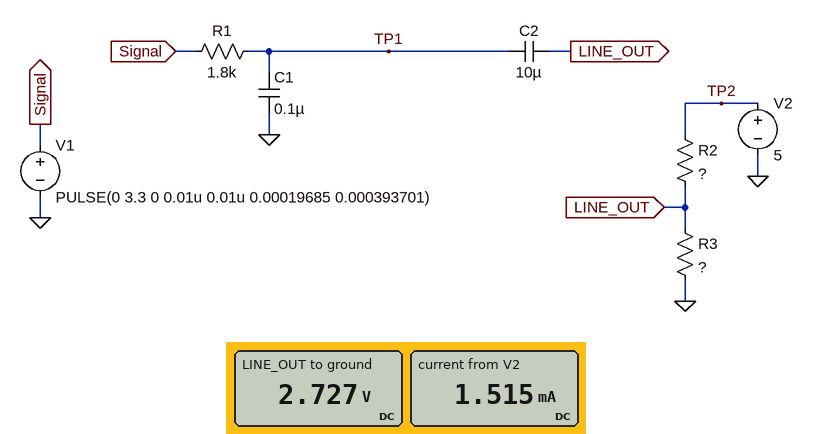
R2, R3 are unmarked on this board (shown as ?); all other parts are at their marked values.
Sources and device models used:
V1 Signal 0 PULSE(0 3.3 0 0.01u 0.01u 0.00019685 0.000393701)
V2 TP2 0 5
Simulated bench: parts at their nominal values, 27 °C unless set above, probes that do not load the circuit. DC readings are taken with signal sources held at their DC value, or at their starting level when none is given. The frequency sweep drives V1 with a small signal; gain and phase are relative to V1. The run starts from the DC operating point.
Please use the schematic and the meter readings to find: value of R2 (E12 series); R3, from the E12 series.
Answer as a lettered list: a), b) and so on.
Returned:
a) 1.5 kΩ
b) 1.8 kΩ
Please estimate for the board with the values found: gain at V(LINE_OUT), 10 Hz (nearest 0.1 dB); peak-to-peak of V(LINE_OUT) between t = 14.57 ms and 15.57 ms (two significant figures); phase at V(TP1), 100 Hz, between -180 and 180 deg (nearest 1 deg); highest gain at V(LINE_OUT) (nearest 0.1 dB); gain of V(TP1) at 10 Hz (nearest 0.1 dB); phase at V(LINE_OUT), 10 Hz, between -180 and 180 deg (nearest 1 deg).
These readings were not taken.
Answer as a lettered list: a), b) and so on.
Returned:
a) -11.5 dB
b) 970 mV
c) -10 deg
d) -10.2 dB
e) -4.7 dB
f) 31 deg
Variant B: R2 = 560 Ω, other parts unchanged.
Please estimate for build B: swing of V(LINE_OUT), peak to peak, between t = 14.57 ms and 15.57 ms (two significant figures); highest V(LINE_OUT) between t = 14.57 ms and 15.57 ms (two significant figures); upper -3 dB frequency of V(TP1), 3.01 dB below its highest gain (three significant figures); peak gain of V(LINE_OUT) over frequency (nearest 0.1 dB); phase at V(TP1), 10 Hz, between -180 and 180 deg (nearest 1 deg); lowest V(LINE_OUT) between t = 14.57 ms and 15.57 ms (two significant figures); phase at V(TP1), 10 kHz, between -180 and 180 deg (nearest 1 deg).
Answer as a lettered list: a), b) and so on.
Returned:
a) 630 mV
b) 4.3 V
c) 7.37 Hz
d) -14.4 dB
e) -40 deg
f) 3.7 V
g) -65 deg
